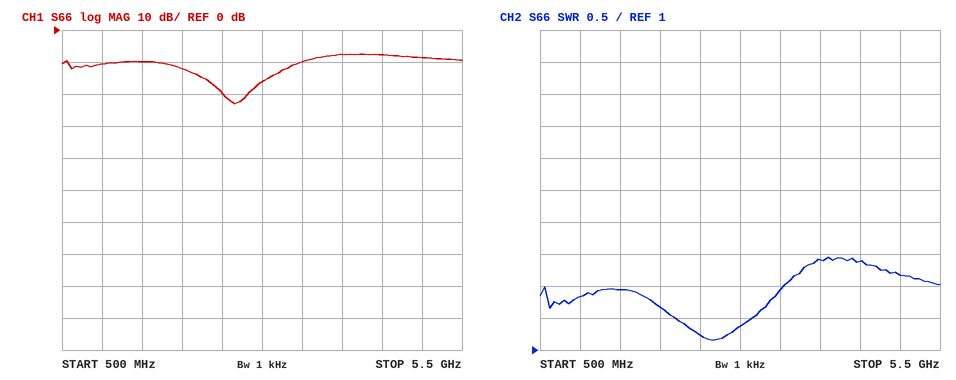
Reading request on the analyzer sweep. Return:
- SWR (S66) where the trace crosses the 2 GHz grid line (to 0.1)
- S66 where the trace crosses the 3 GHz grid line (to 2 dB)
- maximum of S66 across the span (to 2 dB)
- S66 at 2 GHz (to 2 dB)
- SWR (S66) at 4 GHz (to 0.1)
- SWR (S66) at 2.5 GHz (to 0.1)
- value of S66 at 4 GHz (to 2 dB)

1.7
-16 dB
-8 dB
-12 dB
2.4
1.2
-8 dB
